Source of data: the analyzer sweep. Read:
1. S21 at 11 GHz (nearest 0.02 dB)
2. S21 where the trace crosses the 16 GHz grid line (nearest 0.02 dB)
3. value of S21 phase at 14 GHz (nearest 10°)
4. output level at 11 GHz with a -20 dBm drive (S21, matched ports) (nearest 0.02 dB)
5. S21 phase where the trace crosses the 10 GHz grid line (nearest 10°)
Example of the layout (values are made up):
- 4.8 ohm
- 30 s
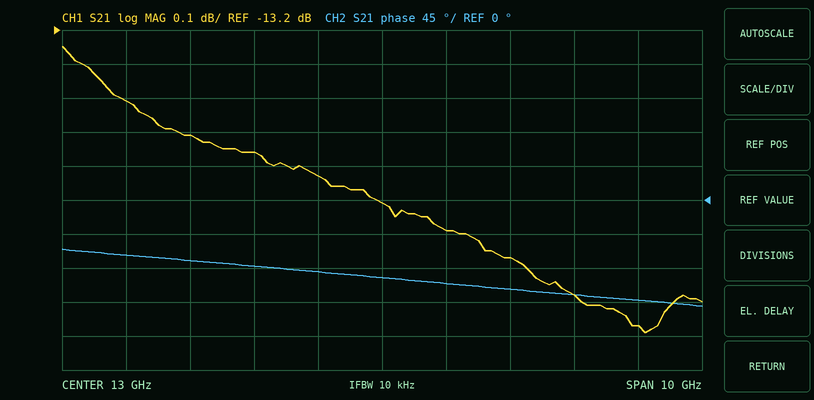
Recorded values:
- -13.56 dB
- -13.98 dB
- -110°
- -33.56 dBm
- -80°
